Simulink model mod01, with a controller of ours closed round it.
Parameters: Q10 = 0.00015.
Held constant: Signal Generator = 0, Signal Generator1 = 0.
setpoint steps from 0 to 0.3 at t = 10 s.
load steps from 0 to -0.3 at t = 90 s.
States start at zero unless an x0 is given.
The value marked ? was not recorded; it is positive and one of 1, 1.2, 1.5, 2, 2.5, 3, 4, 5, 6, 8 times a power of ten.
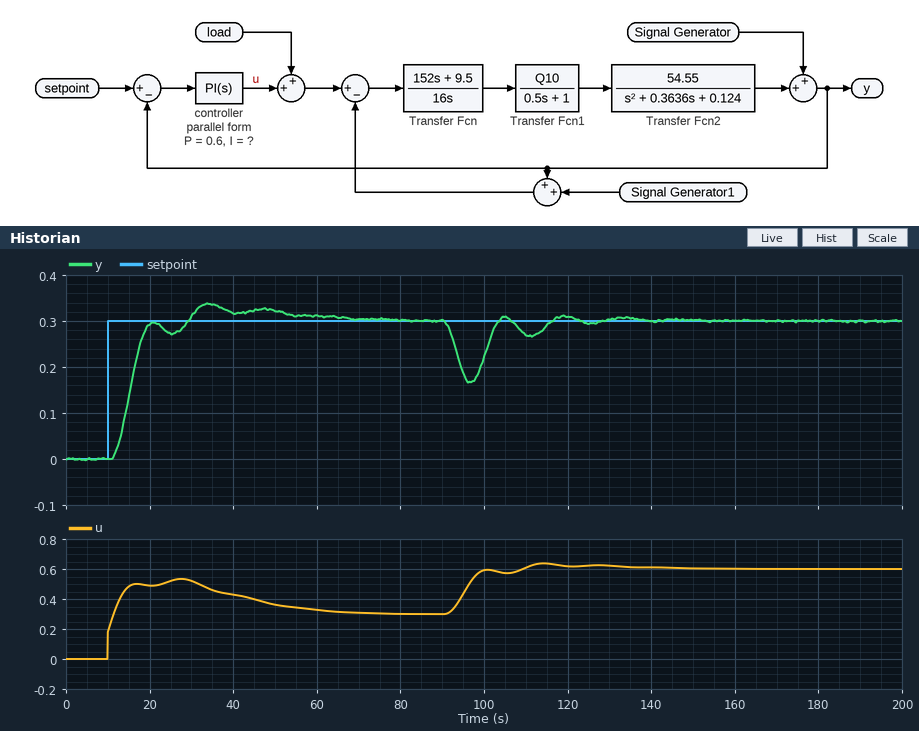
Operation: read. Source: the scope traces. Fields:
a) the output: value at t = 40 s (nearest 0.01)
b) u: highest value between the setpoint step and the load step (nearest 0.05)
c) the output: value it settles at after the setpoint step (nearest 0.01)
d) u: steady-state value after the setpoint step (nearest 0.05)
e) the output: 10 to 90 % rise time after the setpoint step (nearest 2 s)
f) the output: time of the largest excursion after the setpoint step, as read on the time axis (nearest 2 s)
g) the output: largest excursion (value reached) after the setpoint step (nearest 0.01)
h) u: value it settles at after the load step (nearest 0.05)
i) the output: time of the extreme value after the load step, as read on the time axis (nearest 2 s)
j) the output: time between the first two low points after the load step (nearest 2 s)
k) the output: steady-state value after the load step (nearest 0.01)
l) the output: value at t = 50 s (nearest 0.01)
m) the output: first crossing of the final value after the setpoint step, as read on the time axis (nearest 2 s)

0.32
0.55
0.30
0.30
6 s
34 s
0.34
0.60
96 s
14 s
0.30
0.32
30 s
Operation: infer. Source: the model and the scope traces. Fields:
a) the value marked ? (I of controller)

0.3
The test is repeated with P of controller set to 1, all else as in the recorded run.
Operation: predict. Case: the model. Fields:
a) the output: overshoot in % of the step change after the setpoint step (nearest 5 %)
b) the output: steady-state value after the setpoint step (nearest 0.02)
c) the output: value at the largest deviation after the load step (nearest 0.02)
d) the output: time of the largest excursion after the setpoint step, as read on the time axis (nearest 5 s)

10 %
0.30
0.18
30 s
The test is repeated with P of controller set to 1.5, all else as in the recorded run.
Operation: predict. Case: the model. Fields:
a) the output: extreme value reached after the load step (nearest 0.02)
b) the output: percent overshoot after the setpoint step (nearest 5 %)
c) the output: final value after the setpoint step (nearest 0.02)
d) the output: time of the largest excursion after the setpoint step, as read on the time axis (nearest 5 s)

0.18
10 %
0.30
30 s
